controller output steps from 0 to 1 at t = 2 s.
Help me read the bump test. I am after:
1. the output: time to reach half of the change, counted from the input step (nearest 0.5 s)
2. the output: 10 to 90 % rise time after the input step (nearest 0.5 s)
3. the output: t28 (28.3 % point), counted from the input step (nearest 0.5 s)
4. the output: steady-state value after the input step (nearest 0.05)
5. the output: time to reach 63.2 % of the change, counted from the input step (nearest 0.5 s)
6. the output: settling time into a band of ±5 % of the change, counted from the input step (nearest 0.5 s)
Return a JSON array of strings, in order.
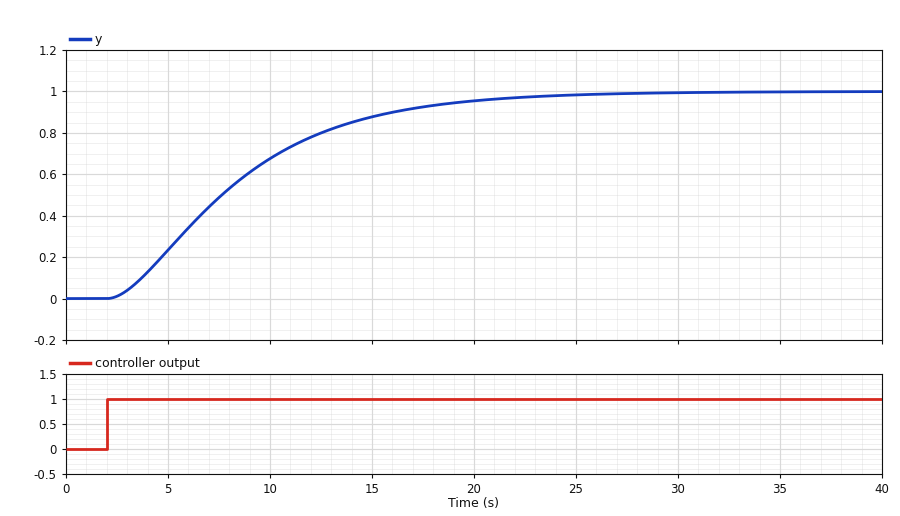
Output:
["5.5 s", "12.5 s", "3.5 s", "1.00", "7.5 s", "17.5 s"]
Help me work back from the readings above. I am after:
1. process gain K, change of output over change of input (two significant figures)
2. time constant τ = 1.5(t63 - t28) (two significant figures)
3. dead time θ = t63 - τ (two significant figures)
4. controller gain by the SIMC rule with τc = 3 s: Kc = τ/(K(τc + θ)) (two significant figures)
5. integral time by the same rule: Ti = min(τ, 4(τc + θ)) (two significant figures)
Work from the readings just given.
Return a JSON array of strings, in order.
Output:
["1.0", "6.0 s", "1.5 s", "1.3", "6.0 s"]
